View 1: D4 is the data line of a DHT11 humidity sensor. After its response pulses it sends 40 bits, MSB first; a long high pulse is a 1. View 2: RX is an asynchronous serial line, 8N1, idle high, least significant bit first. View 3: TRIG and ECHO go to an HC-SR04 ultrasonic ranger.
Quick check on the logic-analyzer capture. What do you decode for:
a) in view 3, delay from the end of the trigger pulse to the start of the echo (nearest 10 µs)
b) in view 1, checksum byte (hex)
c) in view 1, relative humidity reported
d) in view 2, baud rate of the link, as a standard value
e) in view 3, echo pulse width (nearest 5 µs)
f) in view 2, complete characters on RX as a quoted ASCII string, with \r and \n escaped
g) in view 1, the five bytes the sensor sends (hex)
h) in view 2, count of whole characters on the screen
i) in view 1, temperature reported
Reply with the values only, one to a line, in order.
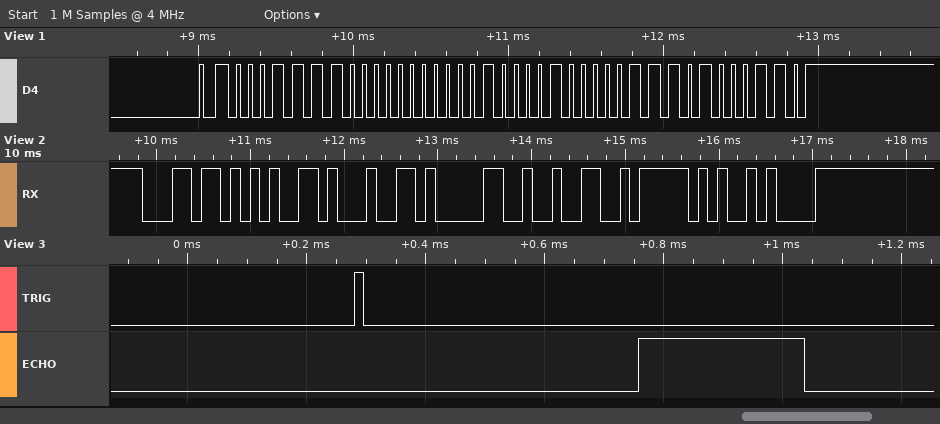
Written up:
460 µs
0x46
30 %
9600 baud
280 µs
"led02_\n"
1E 00 21 07 46
7
33.7 °C
